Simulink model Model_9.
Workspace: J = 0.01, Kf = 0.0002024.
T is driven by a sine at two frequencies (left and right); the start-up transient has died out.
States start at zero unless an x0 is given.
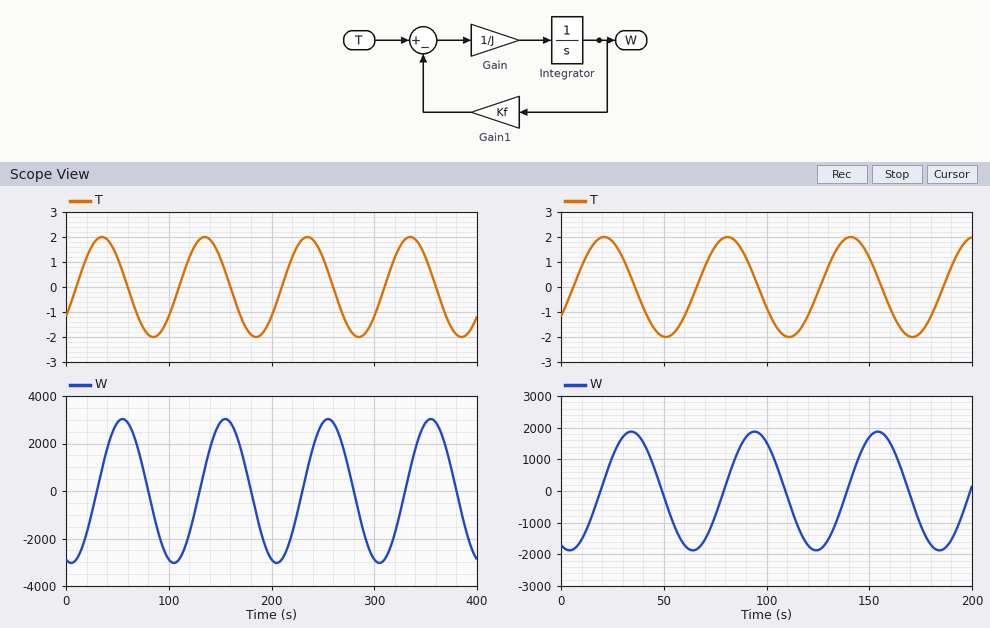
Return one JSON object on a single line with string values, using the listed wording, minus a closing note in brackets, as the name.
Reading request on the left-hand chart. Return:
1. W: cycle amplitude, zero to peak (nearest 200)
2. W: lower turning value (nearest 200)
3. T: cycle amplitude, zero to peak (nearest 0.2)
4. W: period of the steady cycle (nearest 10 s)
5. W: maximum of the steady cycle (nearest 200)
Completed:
{"W: cycle amplitude, zero to peak": "3000", "W: lower turning value": "-3000", "T: cycle amplitude, zero to peak": "2.0", "W: period of the steady cycle": "100 s", "W: maximum of the steady cycle": "3000"}
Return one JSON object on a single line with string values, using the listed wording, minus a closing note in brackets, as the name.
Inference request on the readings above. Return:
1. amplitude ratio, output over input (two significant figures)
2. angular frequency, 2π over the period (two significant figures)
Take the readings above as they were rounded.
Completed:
{"amplitude ratio, output over input": "1500", "angular frequency, 2π over the period": "0.063 rad/s"}
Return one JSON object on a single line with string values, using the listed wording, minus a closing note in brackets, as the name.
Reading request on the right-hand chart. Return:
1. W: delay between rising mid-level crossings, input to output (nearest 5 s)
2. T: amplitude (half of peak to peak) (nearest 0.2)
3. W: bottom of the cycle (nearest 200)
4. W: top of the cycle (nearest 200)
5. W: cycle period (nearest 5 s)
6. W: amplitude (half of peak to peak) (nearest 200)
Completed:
{"W: delay between rising mid-level crossings, input to output": "15 s", "T: amplitude (half of peak to peak)": "2.0", "W: bottom of the cycle": "-1800", "W: top of the cycle": "1800", "W: cycle period": "60 s", "W: amplitude (half of peak to peak)": "1800"}
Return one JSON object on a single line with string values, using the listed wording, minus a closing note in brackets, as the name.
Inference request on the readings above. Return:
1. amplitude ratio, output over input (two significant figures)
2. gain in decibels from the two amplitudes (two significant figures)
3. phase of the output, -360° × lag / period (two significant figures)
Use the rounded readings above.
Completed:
{"amplitude ratio, output over input": "900", "gain in decibels from the two amplitudes": "59 dB", "phase of the output, -360° × lag / period": "-90°"}
